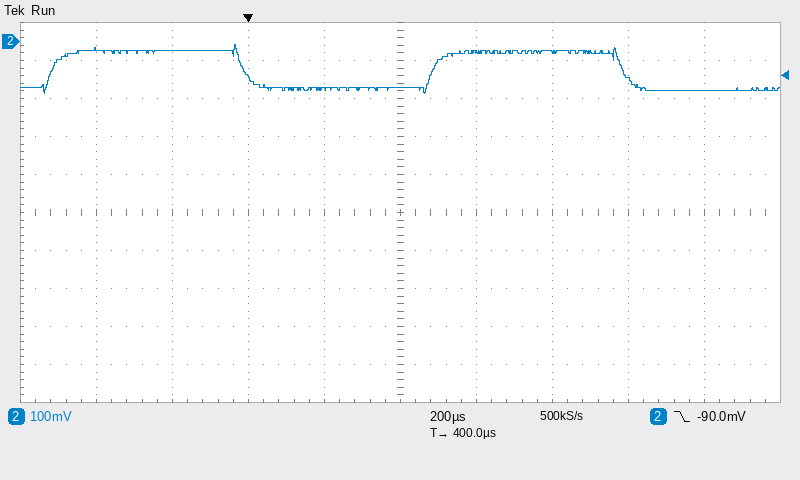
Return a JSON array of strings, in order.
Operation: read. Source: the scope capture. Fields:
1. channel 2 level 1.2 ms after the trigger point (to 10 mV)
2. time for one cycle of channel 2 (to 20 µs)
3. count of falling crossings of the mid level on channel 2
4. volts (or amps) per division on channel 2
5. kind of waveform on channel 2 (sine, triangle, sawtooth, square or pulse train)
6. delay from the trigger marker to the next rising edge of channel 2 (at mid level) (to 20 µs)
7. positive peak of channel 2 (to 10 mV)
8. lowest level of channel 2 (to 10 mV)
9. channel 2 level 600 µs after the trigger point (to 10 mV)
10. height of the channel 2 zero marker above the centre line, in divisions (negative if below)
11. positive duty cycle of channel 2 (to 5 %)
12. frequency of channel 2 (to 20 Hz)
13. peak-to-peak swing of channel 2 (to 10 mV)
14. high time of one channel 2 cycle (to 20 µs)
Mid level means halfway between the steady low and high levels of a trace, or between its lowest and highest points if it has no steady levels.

["-130 mV", "1.00 ms", "2", "100 mV", "square", "480 µs", "-10 mV", "-140 mV", "-30 mV", "+4.5 div", "50 %", "1.00 kHz", "130 mV", "500 µs"]
